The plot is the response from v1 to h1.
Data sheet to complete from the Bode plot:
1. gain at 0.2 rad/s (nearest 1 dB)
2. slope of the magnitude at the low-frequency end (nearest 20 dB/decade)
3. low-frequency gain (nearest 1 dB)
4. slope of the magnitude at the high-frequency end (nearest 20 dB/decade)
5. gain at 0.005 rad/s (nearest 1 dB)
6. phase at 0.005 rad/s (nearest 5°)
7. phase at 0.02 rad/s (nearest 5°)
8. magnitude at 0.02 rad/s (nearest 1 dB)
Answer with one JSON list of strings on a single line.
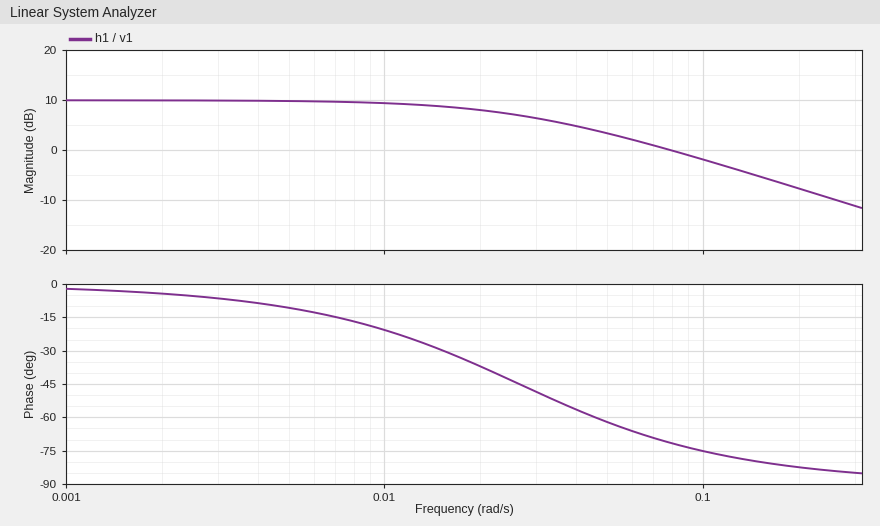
["-8 dB", "0 dB/decade", "10 dB", "-20 dB/decade", "10 dB", "-10°", "-35°", "8 dB"]
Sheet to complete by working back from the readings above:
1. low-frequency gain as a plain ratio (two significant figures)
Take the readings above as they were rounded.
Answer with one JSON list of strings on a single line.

["3.2"]
